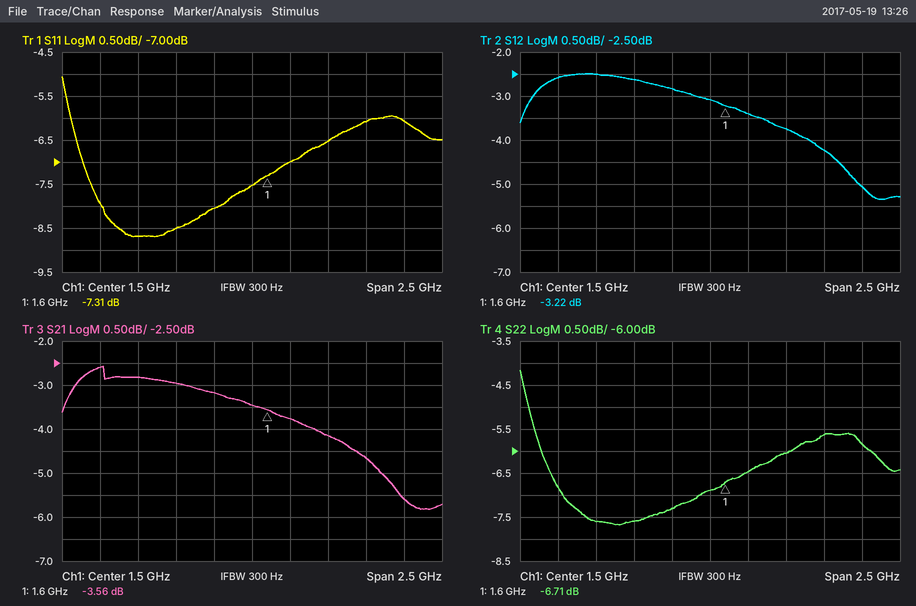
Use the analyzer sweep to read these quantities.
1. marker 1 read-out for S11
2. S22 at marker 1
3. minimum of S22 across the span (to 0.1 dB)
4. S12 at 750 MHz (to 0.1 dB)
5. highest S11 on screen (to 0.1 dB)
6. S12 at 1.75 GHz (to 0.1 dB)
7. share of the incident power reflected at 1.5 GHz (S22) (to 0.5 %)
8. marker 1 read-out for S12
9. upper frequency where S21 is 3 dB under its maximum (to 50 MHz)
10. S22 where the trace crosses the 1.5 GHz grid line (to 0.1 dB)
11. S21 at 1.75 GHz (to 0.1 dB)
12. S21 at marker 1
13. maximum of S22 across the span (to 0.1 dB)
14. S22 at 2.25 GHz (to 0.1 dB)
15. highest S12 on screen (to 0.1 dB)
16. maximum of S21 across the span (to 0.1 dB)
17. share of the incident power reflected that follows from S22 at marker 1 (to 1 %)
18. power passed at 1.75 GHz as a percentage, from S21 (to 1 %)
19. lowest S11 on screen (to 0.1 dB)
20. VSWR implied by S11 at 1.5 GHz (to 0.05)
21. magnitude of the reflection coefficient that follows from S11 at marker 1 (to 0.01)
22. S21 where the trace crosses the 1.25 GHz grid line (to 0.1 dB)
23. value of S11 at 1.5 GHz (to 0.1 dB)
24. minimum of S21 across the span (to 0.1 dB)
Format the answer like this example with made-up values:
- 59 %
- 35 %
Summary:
- -7.31 dB
- -6.71 dB
- -7.7 dB
- -2.5 dB
- -5.1 dB
- -3.4 dB
- 20.5 %
- -3.22 dB
- 2.50 GHz
- -6.9 dB
- -3.8 dB
- -3.56 dB
- -4.2 dB
- -5.6 dB
- -2.5 dB
- -2.6 dB
- 21 %
- 42 %
- -8.7 dB
- 2.45
- 0.43
- -3.2 dB
- -7.5 dB
- -5.8 dB
